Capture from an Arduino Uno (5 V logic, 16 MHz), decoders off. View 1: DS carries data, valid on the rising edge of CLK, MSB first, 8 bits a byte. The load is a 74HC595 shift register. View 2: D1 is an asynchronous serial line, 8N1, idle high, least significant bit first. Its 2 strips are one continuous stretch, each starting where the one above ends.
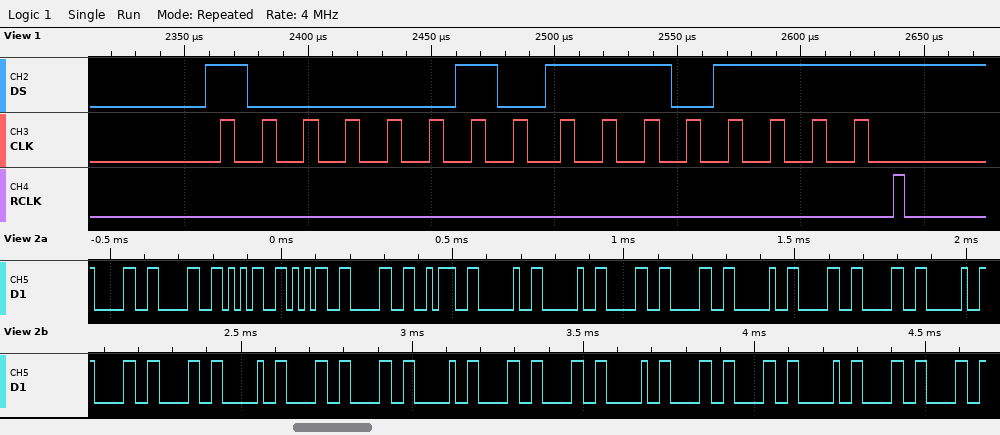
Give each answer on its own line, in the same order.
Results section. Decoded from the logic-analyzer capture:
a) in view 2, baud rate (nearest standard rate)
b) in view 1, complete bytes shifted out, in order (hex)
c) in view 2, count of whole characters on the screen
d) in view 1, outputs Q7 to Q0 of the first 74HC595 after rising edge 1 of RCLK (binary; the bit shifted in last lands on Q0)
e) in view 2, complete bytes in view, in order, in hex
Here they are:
57600 baud
0x82 0xEF
28
11101111
0x30 0x30 0x35 0x35 0x30 0x3A 0x20 0x20 0x30 0x30 0x20 0x30 0x30 0x20 0x30 0x30 0x20 0x30 0x30 0x20 0x30 0x30 0x20 0x30 0x30 0x20 0x30 0x30
